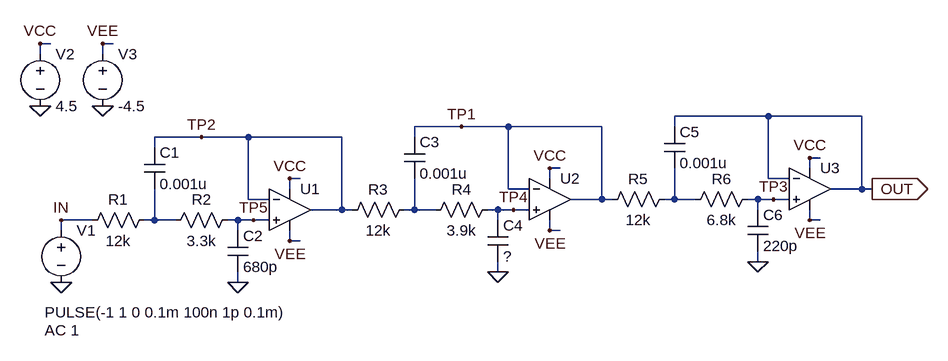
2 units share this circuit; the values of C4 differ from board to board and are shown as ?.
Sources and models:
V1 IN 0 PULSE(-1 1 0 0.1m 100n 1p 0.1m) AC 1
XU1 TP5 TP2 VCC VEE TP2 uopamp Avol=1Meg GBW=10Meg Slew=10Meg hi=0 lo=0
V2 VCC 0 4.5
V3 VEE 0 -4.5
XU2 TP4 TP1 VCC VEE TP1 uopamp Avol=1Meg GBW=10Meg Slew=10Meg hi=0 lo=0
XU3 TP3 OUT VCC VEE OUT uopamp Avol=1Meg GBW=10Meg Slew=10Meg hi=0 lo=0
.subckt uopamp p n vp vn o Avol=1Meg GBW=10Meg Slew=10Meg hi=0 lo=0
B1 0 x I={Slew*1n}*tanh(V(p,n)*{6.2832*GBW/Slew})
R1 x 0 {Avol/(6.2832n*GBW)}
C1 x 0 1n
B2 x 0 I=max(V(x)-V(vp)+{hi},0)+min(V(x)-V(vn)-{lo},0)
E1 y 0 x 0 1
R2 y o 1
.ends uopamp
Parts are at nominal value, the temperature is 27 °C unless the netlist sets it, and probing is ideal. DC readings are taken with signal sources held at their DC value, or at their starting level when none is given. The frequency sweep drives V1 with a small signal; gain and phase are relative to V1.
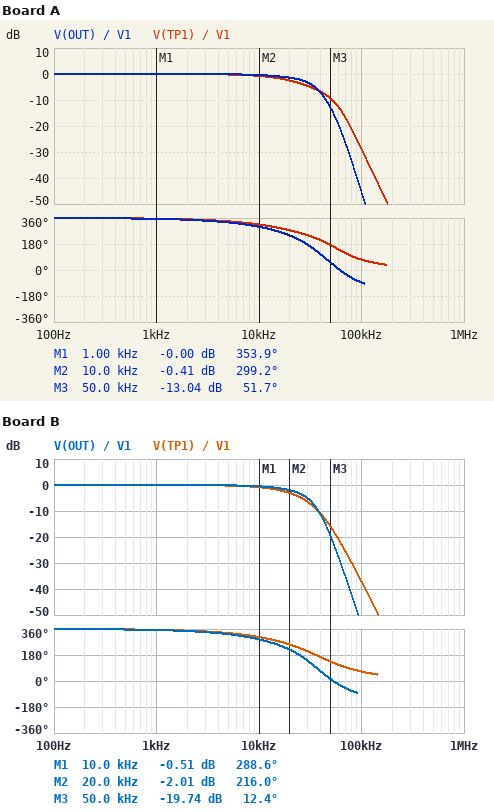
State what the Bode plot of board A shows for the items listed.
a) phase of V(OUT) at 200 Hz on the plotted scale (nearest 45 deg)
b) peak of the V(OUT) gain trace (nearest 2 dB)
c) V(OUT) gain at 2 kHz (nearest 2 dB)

360 deg
0 dB
0 dB
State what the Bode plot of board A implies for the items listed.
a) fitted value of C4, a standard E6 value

150 pF
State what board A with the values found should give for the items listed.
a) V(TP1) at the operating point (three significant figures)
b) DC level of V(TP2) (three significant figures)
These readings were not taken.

-1.00 V
-1.00 V
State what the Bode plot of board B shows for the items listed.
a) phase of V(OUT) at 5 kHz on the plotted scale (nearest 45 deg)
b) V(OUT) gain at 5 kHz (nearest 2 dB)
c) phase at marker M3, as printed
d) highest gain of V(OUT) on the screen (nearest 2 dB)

315 deg
0 dB
12.4 deg
0 dB
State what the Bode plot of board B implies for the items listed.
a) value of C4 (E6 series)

330 pF
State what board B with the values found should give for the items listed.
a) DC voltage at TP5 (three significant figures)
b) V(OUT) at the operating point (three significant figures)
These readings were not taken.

-1.00 V
-1.00 V
